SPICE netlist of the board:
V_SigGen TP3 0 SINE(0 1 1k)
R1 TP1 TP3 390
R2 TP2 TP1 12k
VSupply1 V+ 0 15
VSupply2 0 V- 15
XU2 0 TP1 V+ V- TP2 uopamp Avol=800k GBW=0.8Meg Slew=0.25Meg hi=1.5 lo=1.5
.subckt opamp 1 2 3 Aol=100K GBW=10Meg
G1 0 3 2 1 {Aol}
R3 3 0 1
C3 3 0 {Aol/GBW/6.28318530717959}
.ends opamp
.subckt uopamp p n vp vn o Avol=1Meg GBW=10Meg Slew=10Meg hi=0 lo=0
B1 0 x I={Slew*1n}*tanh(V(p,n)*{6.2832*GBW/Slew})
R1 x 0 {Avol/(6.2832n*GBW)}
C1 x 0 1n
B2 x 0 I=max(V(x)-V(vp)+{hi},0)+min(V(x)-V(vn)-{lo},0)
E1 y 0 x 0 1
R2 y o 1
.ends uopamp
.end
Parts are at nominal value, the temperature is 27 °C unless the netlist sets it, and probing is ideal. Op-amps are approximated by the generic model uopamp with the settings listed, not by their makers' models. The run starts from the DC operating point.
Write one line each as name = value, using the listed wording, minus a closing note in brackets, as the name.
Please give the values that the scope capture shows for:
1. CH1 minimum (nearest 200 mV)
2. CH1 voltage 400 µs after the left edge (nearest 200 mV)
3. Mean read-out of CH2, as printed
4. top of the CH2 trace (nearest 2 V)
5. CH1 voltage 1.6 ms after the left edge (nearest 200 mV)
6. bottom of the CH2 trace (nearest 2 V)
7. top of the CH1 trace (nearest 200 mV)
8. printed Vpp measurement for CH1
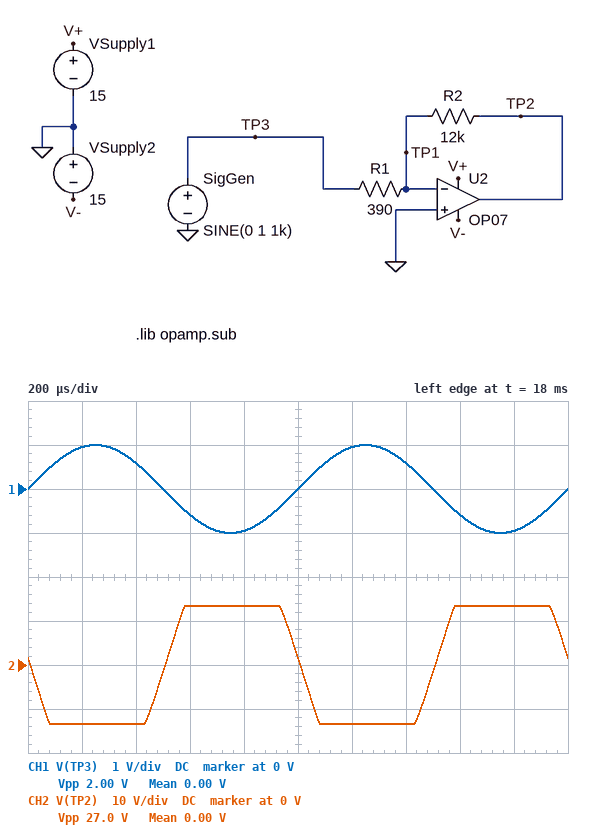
CH1 minimum = -1.0 V
CH1 voltage 400 µs after the left edge = 600 mV
Mean read-out of CH2, as printed = 0.00 V
top of the CH2 trace = 14 V
CH1 voltage 1.6 ms after the left edge = -600 mV
bottom of the CH2 trace = -14 V
top of the CH1 trace = 1.0 V
printed Vpp measurement for CH1 = 2.00 V
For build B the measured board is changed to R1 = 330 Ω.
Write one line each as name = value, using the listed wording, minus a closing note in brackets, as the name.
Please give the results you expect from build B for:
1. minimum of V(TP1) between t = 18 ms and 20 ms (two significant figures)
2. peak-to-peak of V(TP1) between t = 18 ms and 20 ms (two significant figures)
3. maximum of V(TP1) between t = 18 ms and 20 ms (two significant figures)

minimum of V(TP1) between t = 18 ms and 20 ms = -610 mV
peak-to-peak of V(TP1) between t = 18 ms and 20 ms = 1.2 V
maximum of V(TP1) between t = 18 ms and 20 ms = 610 mV
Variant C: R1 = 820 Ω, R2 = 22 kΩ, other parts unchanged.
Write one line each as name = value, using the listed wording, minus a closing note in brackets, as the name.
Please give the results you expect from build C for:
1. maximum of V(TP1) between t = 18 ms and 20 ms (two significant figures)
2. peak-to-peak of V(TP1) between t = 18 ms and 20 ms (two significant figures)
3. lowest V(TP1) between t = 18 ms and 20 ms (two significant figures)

maximum of V(TP1) between t = 18 ms and 20 ms = 480 mV
peak-to-peak of V(TP1) between t = 18 ms and 20 ms = 960 mV
lowest V(TP1) between t = 18 ms and 20 ms = -480 mV
